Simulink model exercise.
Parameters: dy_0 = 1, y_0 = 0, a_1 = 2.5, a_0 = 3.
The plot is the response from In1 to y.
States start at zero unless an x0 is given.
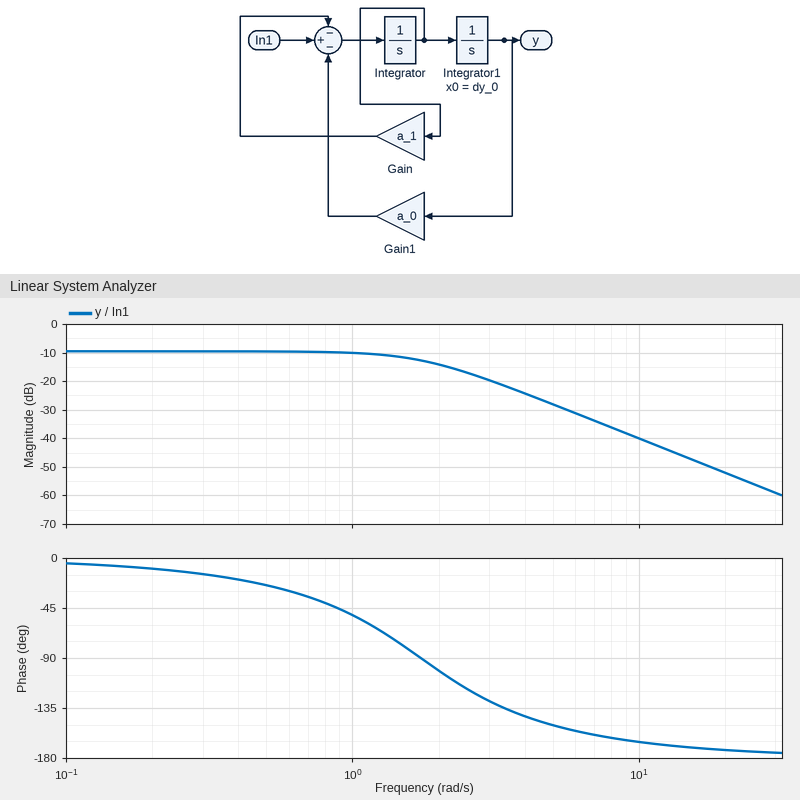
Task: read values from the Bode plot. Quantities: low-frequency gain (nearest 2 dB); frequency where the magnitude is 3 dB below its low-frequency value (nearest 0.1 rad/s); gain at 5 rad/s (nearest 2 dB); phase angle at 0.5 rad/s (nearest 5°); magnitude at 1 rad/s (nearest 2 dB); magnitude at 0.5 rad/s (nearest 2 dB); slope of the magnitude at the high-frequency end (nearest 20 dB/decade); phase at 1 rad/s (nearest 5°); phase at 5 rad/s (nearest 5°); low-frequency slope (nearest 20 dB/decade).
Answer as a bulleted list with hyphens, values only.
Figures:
- -10 dB
- 1.7 rad/s
- -28 dB
- -25°
- -10 dB
- -10 dB
- -40 dB/decade
- -50°
- -150°
- 0 dB/decade
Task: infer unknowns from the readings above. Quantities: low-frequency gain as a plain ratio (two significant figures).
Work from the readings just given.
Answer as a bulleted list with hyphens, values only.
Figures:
- 0.32
